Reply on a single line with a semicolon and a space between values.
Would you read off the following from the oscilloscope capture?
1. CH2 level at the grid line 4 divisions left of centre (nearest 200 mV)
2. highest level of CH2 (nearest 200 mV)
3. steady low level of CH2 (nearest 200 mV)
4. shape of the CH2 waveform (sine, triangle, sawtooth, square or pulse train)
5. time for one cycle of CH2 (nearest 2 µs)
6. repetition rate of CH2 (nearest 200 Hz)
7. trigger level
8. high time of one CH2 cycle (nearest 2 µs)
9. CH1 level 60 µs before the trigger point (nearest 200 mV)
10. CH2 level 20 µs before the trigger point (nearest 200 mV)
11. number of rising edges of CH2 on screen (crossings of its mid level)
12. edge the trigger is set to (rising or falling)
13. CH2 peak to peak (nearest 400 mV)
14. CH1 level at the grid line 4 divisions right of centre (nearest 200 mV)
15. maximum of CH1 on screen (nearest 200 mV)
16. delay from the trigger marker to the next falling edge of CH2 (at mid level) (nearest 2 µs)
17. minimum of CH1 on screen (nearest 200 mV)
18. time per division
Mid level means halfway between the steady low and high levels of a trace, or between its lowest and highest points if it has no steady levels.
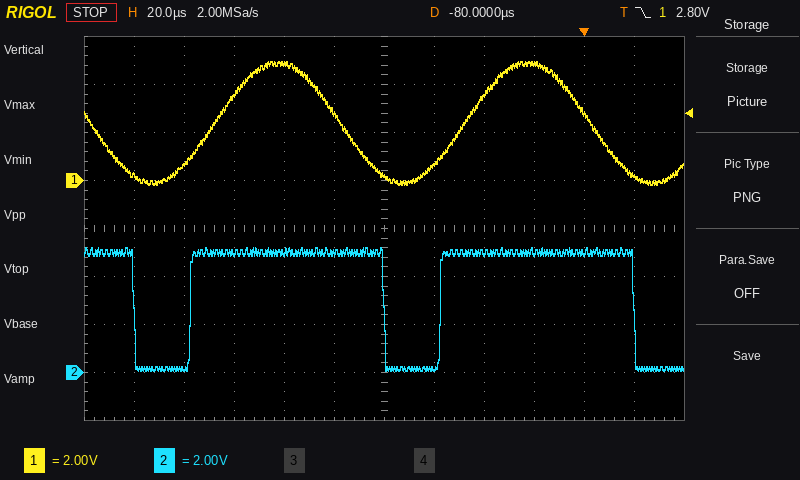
200 mV; 5.2 V; 200 mV; pulse train; 100 µs; 10.0 kHz; 2.80 V; 78 µs; 600 mV; 5.0 V; 2; falling; 5.2 V; 2.8 V; 5.0 V; 20 µs; -200 mV; 20 µs
